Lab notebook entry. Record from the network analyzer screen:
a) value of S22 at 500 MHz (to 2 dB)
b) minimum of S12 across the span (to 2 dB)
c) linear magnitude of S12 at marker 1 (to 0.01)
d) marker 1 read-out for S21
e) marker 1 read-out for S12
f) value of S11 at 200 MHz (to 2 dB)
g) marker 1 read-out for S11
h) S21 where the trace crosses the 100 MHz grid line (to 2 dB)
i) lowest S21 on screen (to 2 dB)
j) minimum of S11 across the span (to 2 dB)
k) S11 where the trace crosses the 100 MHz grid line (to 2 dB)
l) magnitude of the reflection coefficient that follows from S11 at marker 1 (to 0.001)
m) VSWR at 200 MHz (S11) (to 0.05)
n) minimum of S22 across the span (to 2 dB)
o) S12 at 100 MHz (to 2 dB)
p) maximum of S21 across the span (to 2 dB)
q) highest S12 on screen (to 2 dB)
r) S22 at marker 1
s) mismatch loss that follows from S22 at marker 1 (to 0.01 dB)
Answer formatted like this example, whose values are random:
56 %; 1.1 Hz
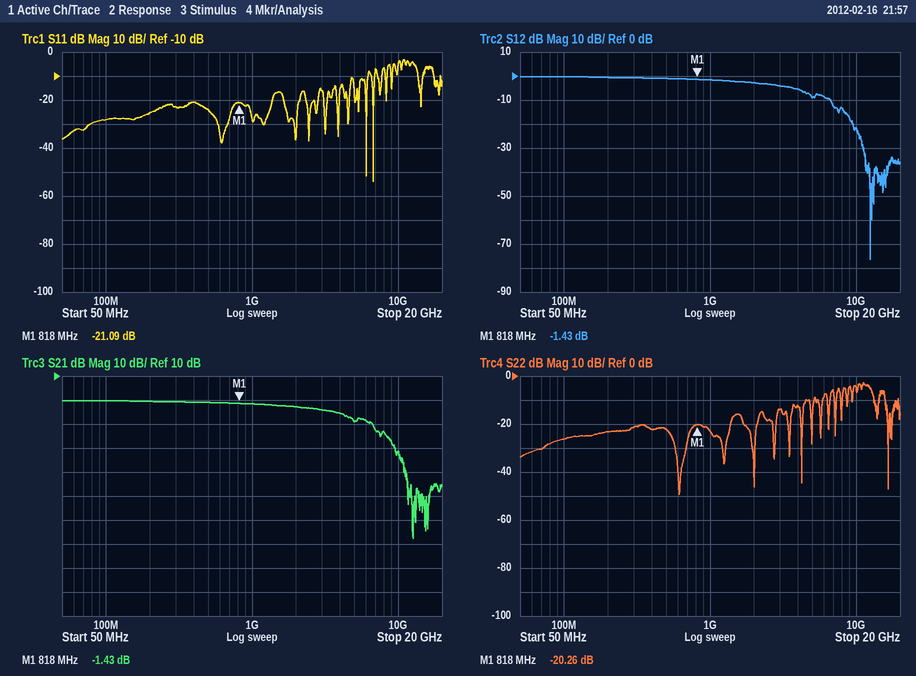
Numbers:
-22 dB; -76 dB; 0.85; -1.43 dB; -1.43 dB; -26 dB; -21.09 dB; 0 dB; -58 dB; -54 dB; -28 dB; 0.088; 1.10; -50 dB; 0 dB; 0 dB; 0 dB; -20.26 dB; 0.04 dB
